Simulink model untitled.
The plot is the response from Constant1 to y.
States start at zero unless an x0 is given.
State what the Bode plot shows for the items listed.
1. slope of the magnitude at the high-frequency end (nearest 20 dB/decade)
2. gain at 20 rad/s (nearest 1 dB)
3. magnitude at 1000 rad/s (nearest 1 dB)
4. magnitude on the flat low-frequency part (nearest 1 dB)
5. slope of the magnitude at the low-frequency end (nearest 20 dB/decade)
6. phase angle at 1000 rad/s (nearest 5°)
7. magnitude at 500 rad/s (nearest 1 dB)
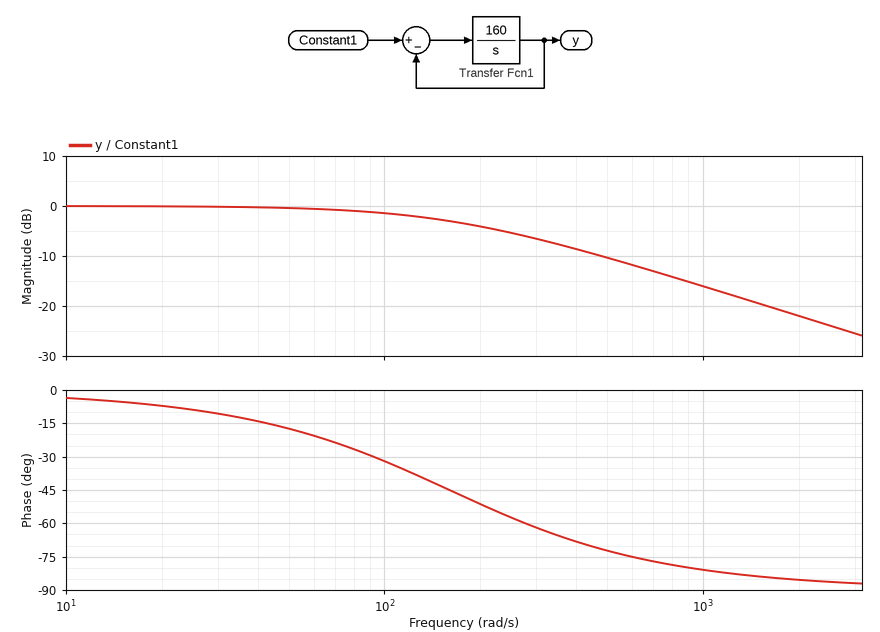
-20 dB/decade
0 dB
-16 dB
0 dB
0 dB/decade
-80°
-10 dB
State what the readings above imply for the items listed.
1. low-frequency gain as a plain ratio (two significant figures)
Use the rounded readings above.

1.0
